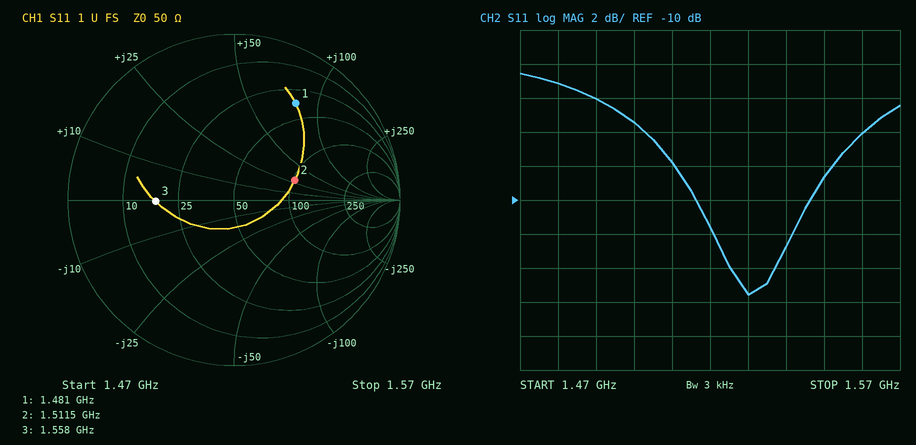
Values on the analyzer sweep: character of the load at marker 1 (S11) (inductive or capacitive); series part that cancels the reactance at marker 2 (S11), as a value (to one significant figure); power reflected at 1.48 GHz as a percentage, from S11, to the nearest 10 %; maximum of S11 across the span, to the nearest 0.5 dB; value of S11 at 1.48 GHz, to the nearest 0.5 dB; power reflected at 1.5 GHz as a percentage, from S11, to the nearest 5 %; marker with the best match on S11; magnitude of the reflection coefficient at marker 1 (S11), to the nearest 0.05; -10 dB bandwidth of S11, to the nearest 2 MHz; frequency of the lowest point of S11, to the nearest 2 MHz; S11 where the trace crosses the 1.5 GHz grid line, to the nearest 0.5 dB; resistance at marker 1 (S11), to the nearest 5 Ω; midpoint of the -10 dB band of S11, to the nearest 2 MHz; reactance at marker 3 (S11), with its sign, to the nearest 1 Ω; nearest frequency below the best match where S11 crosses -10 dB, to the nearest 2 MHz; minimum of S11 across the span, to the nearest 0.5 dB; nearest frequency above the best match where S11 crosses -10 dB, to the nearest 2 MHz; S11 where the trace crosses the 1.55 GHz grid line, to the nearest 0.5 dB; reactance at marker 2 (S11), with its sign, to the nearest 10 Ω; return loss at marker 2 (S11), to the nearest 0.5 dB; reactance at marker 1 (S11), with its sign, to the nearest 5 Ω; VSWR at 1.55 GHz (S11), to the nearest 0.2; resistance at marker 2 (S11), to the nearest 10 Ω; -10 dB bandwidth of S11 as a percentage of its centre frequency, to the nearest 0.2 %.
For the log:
inductive
4 pF
50 %
-2.5 dB
-3.0 dB
30 %
marker 2
0.70
30 MHz
1.530 GHz
-5.5 dB
35 Ω
1.532 GHz
0 Ω
1.516 GHz
-15.5 dB
1.546 GHz
-8.5 dB
+30 Ω
8.5 dB
+80 Ω
2.2
100 Ω
2.0 %
